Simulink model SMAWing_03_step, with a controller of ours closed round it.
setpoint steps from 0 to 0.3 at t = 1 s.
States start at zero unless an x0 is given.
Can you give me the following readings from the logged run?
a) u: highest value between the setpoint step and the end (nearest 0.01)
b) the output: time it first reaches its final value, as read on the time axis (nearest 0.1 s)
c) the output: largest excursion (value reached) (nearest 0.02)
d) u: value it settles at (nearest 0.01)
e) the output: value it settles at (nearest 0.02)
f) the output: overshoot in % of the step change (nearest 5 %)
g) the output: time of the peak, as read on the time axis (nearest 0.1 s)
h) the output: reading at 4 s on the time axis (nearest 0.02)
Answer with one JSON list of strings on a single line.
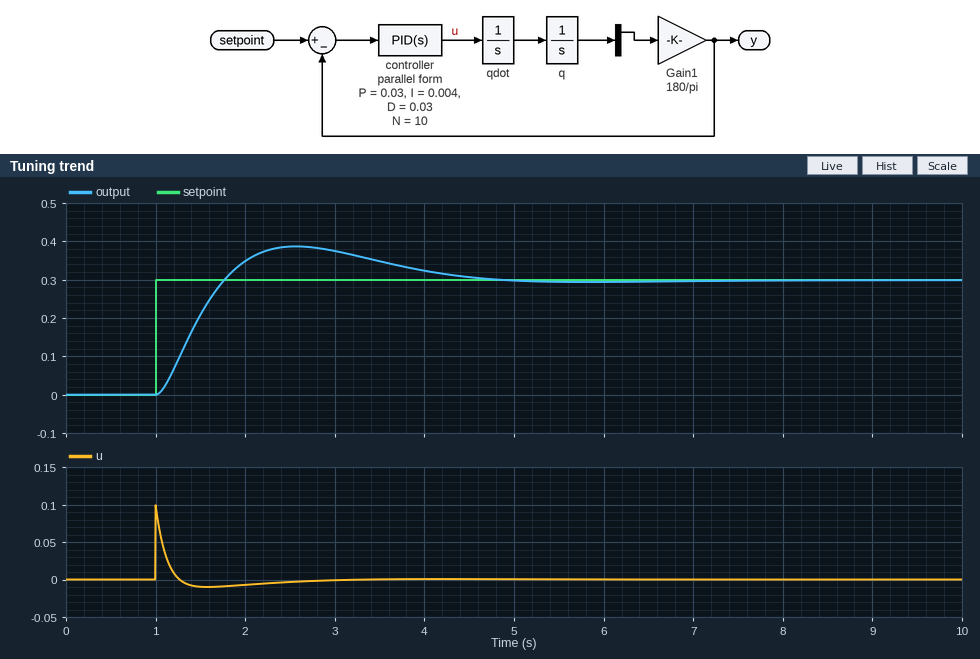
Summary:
["0.10", "1.8 s", "0.38", "0.00", "0.30", "30 %", "2.6 s", "0.32"]
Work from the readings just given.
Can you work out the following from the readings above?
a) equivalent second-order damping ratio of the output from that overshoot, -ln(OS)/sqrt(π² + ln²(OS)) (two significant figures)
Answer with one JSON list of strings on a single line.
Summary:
["0.36"]
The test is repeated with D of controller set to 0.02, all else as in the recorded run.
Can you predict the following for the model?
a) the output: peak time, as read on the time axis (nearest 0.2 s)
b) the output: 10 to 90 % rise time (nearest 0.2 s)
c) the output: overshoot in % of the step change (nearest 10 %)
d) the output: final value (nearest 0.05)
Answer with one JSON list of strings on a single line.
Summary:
["2.8 s", "0.6 s", "40 %", "0.30"]
